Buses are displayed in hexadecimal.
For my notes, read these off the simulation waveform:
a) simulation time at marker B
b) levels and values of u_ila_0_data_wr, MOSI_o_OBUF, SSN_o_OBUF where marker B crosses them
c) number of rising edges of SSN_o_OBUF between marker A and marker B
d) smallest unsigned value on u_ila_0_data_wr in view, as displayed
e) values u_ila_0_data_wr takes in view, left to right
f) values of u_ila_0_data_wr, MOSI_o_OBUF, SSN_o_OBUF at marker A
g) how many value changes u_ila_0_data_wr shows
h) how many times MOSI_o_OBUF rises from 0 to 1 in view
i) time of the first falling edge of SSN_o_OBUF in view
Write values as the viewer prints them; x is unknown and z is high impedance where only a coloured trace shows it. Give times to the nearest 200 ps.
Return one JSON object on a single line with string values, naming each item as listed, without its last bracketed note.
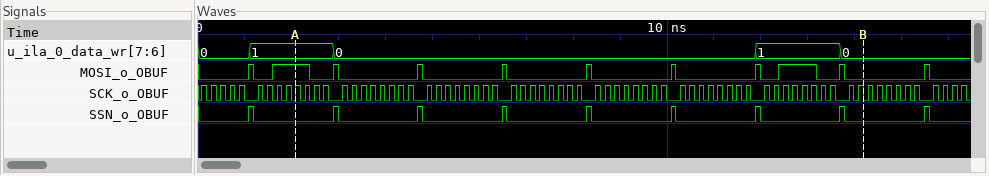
{"simulation time at marker B": "14200 ps", "levels and values of u_ila_0_data_wr, MOSI_o_OBUF, SSN_o_OBUF where marker B crosses them": "u_ila_0_data_wr=0, MOSI_o_OBUF=0, SSN_o_OBUF=0", "number of rising edges of SSN_o_OBUF between marker A and marker B": "7", "smallest unsigned value on u_ila_0_data_wr in view, as displayed": "0", "values u_ila_0_data_wr takes in view, left to right": "0, 1, 0, 1, 0", "values of u_ila_0_data_wr, MOSI_o_OBUF, SSN_o_OBUF at marker A": "u_ila_0_data_wr=1, MOSI_o_OBUF=1, SSN_o_OBUF=0", "how many value changes u_ila_0_data_wr shows": "4", "how many times MOSI_o_OBUF rises from 0 to 1 in view": "11", "time of the first falling edge of SSN_o_OBUF in view": "1200 ps"}
